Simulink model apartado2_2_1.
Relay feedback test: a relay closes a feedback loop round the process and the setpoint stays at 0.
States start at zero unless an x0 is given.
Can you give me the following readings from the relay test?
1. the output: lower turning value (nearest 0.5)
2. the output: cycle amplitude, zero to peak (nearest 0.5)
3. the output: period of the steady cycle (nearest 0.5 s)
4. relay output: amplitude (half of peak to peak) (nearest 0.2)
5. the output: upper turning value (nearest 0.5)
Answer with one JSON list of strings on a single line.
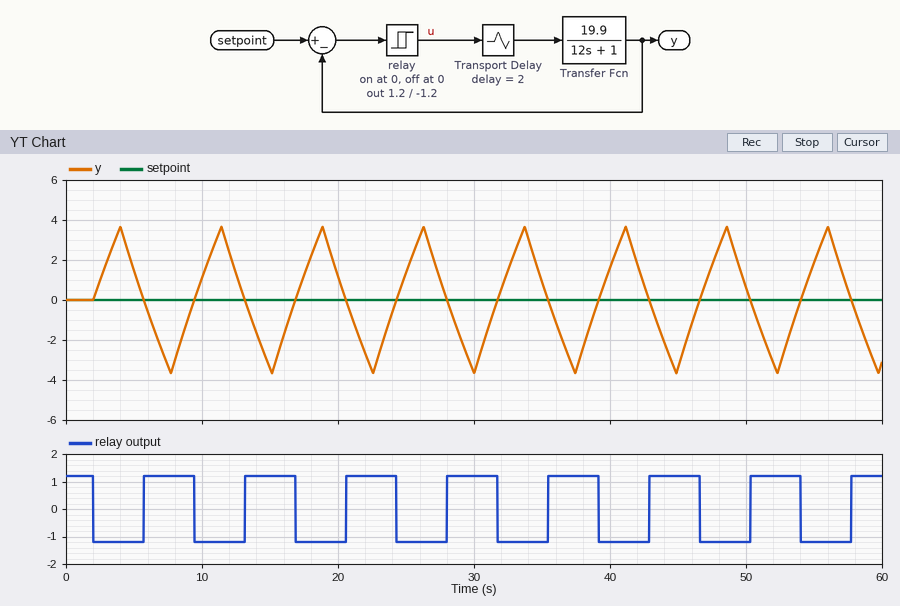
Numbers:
["-3.5", "3.5", "7.5 s", "1.2", "3.5"]
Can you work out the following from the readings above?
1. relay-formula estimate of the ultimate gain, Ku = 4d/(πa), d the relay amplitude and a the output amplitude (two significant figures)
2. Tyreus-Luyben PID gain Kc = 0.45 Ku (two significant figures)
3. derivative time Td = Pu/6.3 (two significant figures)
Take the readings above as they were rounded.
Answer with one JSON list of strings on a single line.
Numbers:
["0.44", "0.20", "1.2 s"]
